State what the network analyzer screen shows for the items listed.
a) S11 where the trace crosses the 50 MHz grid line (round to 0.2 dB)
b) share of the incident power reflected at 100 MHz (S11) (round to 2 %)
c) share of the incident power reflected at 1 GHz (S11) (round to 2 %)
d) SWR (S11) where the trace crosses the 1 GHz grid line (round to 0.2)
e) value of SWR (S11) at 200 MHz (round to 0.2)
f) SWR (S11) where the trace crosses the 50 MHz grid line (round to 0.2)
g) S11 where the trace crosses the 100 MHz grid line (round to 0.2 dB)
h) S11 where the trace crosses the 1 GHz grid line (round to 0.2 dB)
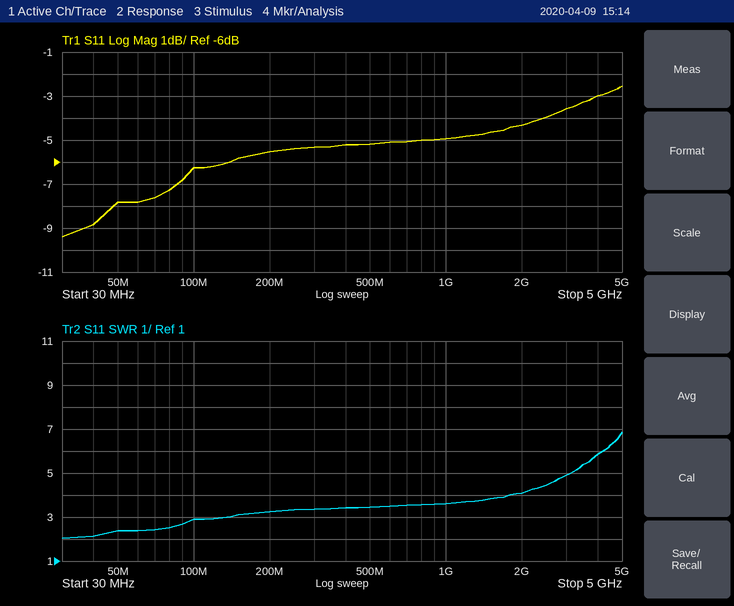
-7.8 dB
24 %
32 %
3.6
3.2
2.4
-6.2 dB
-5.0 dB
